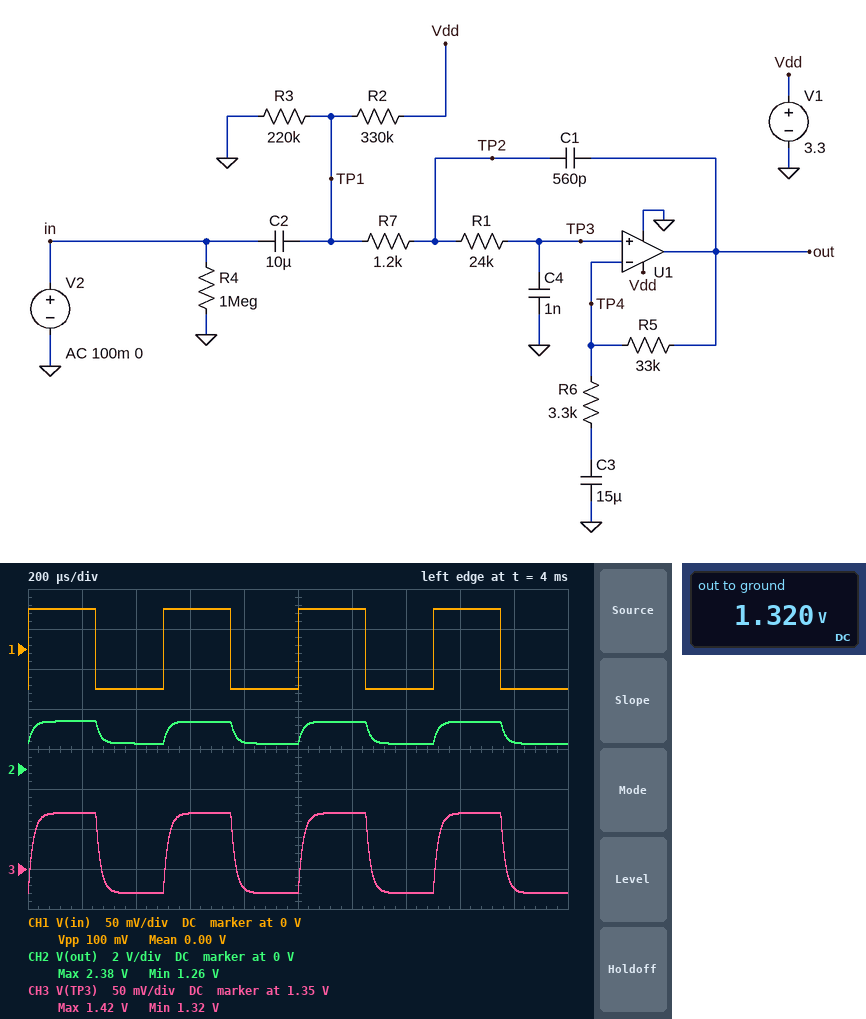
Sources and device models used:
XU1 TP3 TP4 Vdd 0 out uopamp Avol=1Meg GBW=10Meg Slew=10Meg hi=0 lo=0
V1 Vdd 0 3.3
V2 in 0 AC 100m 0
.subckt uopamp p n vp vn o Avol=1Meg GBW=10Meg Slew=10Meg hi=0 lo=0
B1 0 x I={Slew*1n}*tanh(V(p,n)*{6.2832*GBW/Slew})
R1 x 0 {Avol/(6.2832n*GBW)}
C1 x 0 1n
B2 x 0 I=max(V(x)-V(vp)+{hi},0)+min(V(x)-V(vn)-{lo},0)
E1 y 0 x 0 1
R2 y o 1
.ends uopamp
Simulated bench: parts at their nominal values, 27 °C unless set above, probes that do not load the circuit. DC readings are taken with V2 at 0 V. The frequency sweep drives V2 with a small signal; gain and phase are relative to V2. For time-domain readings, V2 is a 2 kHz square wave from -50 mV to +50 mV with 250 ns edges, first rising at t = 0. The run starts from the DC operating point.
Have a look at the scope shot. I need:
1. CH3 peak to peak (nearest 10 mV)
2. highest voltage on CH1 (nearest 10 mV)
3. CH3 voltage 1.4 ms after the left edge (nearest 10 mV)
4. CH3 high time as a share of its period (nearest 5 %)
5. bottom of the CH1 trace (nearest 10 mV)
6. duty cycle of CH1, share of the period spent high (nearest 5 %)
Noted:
100 mV
50 mV
1.32 V
50 %
-50 mV
50 %
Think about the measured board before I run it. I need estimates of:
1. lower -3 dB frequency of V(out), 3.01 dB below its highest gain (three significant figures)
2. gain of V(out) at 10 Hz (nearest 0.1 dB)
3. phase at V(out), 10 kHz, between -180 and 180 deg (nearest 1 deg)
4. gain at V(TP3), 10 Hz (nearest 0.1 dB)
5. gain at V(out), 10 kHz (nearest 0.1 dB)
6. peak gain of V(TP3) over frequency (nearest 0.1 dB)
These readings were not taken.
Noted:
3.19 Hz
20.4 dB
-52 deg
0 dB
17.4 dB
0 dB
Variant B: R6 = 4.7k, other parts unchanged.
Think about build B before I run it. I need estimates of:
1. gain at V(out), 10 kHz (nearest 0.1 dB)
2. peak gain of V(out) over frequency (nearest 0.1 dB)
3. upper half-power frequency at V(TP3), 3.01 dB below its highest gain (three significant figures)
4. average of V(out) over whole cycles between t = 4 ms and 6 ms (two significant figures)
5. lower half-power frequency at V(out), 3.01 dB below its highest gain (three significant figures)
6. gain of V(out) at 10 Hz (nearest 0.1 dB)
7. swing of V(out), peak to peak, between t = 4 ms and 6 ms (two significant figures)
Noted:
14.1 dB
18.1 dB
8.09 kHz
1.7 V
2.23 Hz
17.9 dB
810 mV
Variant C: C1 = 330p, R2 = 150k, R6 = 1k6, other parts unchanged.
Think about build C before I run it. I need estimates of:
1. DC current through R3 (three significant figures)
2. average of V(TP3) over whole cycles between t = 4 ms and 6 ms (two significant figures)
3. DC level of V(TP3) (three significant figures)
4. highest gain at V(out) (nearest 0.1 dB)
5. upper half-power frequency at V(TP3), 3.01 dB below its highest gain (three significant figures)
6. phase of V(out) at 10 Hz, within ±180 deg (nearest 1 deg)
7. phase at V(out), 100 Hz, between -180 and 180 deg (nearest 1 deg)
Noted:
8.92 µA
2.0 V
1.96 V
26.7 dB
9.76 kHz
33 deg
3 deg
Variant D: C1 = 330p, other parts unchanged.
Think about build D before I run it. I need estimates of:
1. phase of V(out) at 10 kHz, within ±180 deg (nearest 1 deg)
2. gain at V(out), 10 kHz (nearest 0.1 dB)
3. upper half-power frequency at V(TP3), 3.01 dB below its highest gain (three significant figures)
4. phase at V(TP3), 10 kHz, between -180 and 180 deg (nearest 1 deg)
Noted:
-55 deg
16.5 dB
7.67 kHz
-54 deg
